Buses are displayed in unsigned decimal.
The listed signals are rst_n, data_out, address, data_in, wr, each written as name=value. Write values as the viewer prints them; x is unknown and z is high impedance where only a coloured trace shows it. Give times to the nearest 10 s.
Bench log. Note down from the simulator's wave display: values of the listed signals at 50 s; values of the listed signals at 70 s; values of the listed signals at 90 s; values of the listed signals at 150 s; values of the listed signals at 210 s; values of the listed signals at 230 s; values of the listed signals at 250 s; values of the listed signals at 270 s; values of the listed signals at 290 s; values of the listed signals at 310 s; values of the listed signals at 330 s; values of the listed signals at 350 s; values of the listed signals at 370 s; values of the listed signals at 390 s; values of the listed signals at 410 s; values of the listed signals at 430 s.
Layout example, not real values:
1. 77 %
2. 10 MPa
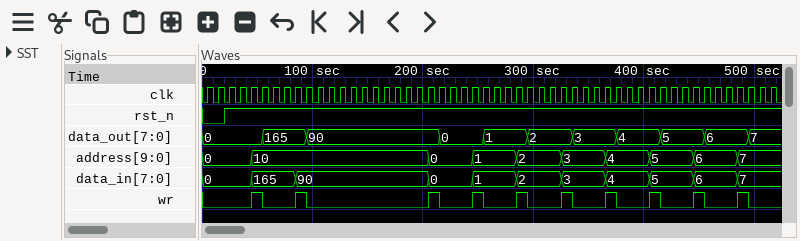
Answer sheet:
1. rst_n=1, data_out=0, address=10, data_in=165, wr=1
2. rst_n=1, data_out=165, address=10, data_in=165, wr=0
3. rst_n=1, data_out=165, address=10, data_in=90, wr=1
4. rst_n=1, data_out=90, address=10, data_in=90, wr=0
5. rst_n=1, data_out=90, address=0, data_in=0, wr=1
6. rst_n=1, data_out=0, address=0, data_in=0, wr=0
7. rst_n=1, data_out=0, address=1, data_in=1, wr=1
8. rst_n=1, data_out=1, address=1, data_in=1, wr=0
9. rst_n=1, data_out=1, address=2, data_in=2, wr=1
10. rst_n=1, data_out=2, address=2, data_in=2, wr=0
11. rst_n=1, data_out=2, address=3, data_in=3, wr=1
12. rst_n=1, data_out=3, address=3, data_in=3, wr=0
13. rst_n=1, data_out=3, address=4, data_in=4, wr=1
14. rst_n=1, data_out=4, address=4, data_in=4, wr=0
15. rst_n=1, data_out=4, address=5, data_in=5, wr=1
16. rst_n=1, data_out=5, address=5, data_in=5, wr=0
